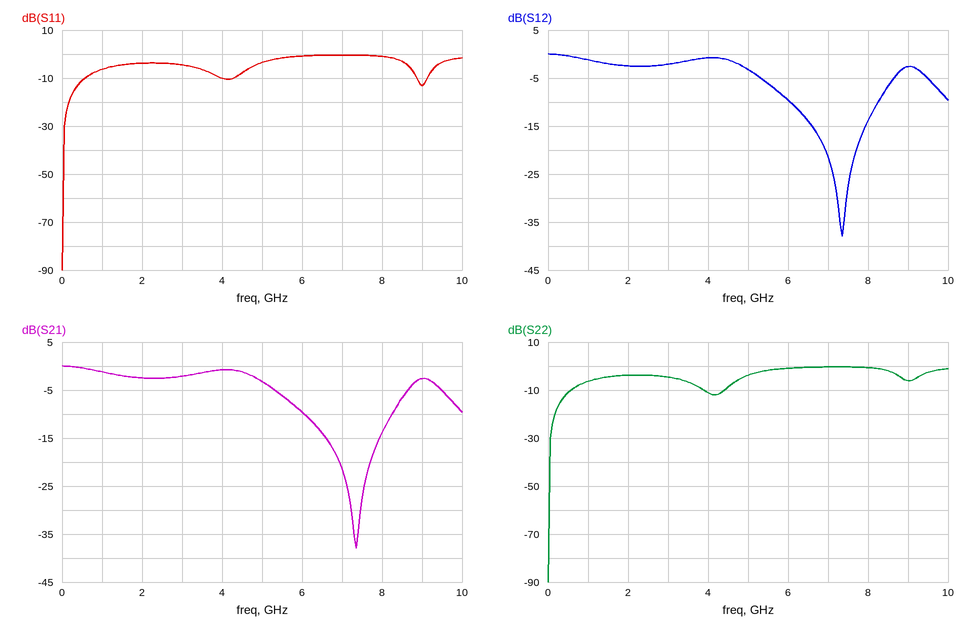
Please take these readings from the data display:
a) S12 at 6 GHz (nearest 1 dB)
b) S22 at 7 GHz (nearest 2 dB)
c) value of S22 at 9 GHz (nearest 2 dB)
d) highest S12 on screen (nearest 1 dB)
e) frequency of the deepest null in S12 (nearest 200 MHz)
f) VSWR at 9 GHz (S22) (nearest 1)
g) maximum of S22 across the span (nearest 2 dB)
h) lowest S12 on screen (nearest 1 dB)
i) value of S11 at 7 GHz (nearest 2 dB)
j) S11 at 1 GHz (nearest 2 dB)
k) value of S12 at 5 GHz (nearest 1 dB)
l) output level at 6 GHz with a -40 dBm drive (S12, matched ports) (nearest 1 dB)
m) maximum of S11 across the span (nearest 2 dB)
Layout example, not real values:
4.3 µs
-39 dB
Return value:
-10 dB
0 dB
-6 dB
0 dB
7.4 GHz
3
0 dB
-38 dB
0 dB
-6 dB
-3 dB
-50 dBm
0 dB
